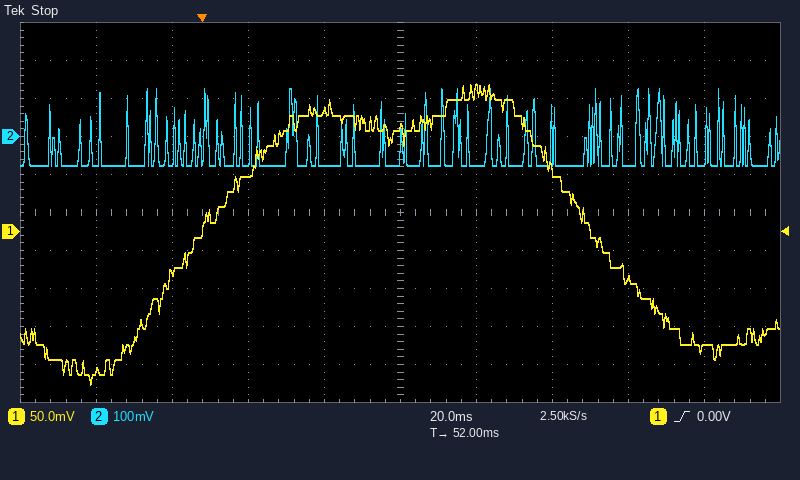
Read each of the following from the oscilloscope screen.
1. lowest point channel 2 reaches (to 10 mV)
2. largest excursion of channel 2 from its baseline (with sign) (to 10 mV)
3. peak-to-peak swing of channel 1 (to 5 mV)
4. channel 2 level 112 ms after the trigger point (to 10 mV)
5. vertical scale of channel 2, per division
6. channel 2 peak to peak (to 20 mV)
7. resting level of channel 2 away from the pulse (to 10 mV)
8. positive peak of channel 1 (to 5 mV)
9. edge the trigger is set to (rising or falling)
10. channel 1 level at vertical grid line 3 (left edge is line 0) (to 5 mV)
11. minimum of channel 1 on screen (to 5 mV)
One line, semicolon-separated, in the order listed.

-80 mV; +200 mV; 395 mV; -80 mV; 100 mV; 200 mV; -80 mV; 195 mV; rising; 75 mV; -200 mV
